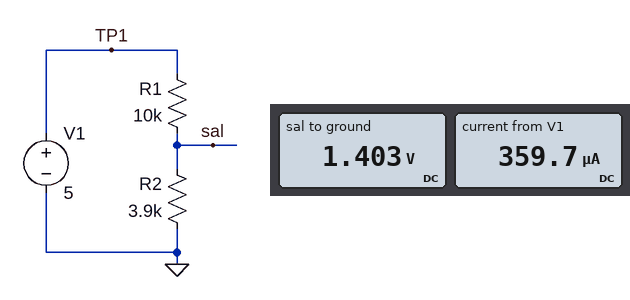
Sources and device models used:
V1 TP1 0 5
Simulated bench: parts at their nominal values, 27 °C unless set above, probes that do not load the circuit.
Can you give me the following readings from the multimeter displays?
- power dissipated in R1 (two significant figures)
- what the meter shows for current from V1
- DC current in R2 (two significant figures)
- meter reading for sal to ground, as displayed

1.3 mW
359.7 µA
360 µA
1.403 V
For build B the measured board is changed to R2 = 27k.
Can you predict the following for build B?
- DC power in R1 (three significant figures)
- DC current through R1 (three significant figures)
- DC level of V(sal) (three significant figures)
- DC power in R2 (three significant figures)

183 µW
135 µA
3.65 V
493 µW
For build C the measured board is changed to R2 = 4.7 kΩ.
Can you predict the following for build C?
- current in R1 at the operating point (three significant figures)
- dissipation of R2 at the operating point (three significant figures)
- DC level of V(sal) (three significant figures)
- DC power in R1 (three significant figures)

340 µA
544 µW
1.60 V
1.16 mW
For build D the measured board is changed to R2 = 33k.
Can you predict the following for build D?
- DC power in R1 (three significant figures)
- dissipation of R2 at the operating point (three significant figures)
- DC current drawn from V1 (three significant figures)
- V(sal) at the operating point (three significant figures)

135 µW
446 µW
116 µA
3.84 V
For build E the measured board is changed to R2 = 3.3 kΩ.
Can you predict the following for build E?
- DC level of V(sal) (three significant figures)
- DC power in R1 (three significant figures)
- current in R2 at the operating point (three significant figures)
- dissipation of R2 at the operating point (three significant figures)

1.24 V
1.41 mW
376 µA
466 µW
